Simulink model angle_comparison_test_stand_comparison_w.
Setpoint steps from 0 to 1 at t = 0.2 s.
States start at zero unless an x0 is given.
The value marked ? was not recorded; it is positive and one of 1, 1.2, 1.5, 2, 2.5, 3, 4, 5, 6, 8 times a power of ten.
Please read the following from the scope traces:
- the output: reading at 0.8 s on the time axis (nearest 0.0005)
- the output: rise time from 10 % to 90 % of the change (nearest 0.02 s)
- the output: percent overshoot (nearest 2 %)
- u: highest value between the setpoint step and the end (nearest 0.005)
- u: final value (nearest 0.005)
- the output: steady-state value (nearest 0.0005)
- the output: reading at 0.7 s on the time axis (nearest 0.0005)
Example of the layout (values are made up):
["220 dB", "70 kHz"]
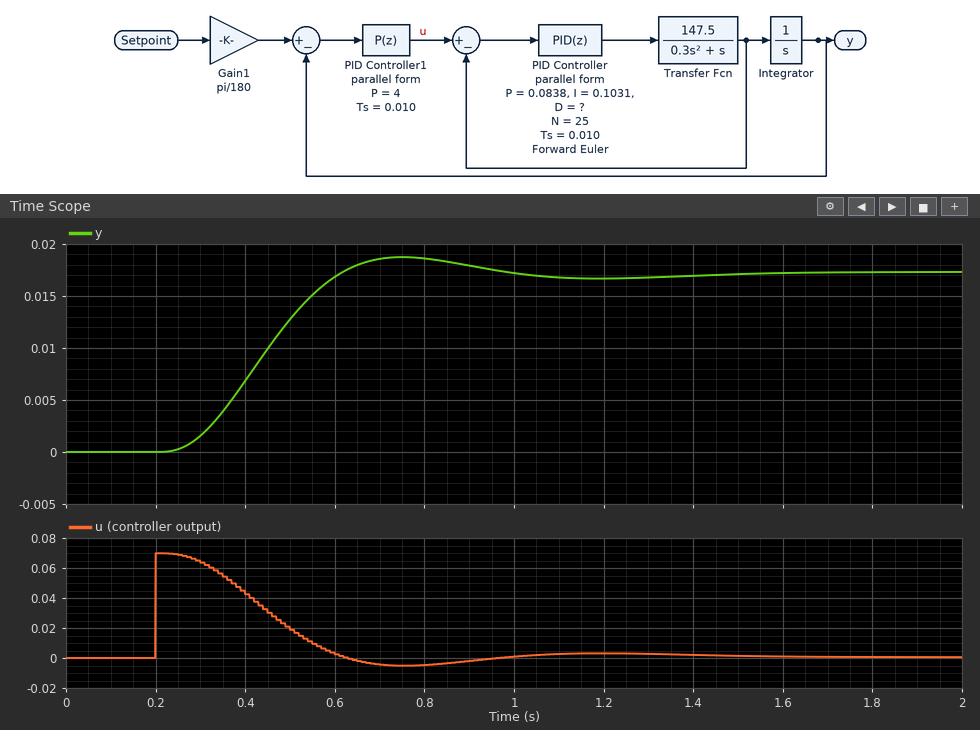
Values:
["0.0185", "0.26 s", "8 %", "0.070", "0.000", "0.0175", "0.0185"]
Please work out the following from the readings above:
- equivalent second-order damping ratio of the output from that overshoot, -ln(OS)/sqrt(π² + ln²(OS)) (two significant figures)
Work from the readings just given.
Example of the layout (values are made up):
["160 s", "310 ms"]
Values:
["0.63"]
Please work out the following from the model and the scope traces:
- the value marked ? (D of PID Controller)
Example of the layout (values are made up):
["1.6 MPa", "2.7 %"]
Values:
["0.015"]
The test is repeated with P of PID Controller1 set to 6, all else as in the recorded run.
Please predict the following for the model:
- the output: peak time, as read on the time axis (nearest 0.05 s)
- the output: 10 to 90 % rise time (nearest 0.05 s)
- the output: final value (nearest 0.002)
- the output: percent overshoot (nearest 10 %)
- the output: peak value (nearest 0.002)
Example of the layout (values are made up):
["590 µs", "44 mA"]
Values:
["0.65 s", "0.20 s", "0.018", "20 %", "0.022"]
